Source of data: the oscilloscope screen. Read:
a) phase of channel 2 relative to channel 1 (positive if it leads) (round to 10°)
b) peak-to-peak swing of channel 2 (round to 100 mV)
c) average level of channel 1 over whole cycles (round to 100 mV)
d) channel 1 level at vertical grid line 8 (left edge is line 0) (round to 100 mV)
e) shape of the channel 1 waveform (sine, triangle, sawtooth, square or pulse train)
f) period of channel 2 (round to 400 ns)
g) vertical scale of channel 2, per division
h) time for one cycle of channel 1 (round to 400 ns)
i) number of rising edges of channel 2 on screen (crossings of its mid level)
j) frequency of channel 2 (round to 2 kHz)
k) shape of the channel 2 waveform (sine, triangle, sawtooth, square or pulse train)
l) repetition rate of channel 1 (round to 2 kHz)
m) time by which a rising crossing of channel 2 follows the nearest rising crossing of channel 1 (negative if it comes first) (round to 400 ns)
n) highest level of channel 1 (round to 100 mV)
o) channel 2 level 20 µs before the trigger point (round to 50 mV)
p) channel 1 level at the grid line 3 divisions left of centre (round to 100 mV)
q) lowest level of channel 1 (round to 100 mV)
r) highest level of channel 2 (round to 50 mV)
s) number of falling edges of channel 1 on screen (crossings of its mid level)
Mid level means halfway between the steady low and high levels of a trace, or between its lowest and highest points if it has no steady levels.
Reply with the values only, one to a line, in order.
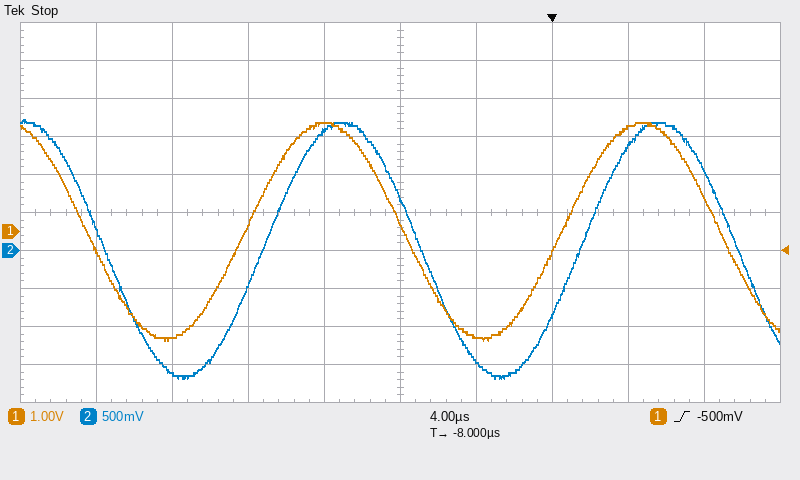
-20°
3.40 V
0.0 V
2.7 V
sine
16.8 µs
500 mV
16.8 µs
2
60 kHz
sine
60 kHz
+800 ns
2.9 V
-1.60 V
-2.8 V
-2.9 V
1.70 V
3
